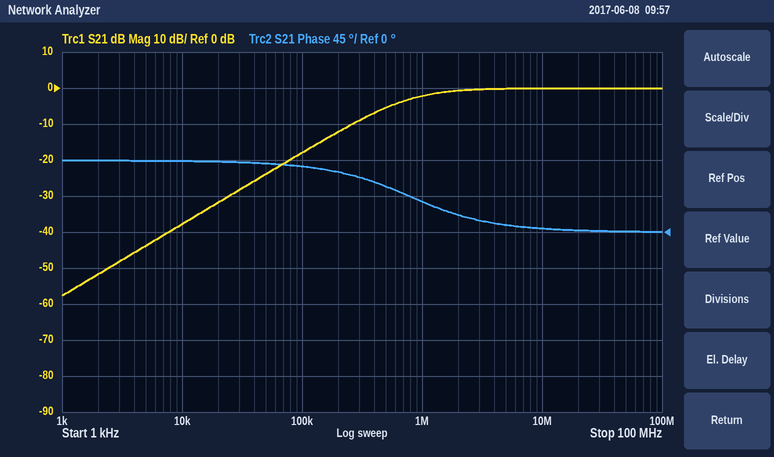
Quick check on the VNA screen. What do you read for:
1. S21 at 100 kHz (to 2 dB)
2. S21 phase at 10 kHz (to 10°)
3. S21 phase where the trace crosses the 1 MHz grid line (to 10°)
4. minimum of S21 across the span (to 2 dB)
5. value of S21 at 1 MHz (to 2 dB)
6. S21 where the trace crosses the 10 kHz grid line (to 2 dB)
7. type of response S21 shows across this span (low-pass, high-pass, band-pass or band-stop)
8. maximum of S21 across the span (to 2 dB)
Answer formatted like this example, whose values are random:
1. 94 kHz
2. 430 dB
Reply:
1. -18 dB
2. 90°
3. 40°
4. -58 dB
5. -2 dB
6. -38 dB
7. high-pass
8. 0 dB
